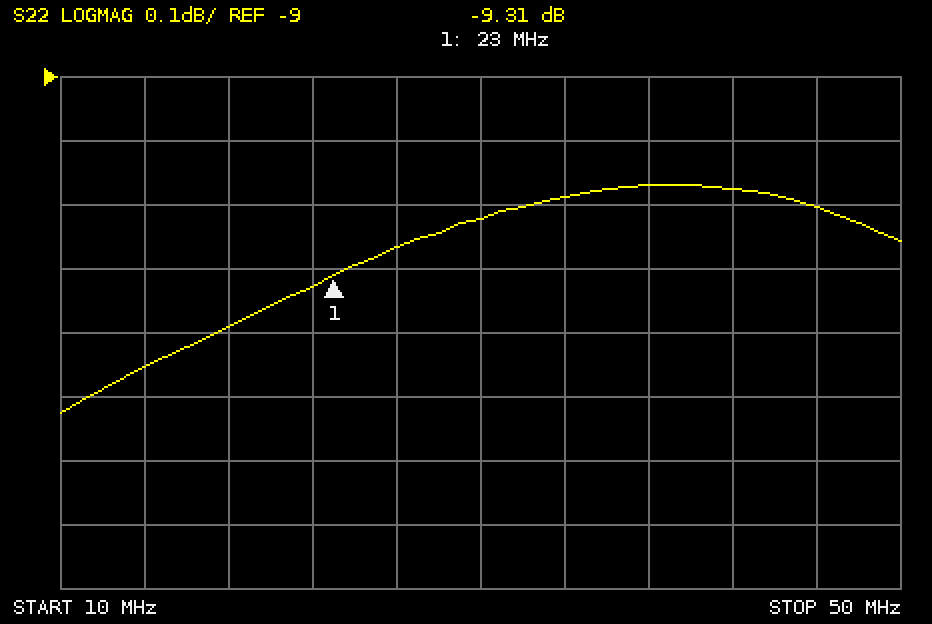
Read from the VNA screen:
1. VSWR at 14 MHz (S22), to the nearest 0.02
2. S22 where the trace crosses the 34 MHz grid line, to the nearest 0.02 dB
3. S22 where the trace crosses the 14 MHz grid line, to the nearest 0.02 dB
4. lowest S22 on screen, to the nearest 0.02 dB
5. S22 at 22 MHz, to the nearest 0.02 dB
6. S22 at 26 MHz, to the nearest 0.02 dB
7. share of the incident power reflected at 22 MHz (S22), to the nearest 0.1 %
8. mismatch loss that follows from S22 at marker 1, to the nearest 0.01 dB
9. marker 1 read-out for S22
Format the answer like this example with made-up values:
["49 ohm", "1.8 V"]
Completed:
["2.02", "-9.18 dB", "-9.46 dB", "-9.52 dB", "-9.32 dB", "-9.26 dB", "11.7 %", "0.54 dB", "-9.31 dB"]
